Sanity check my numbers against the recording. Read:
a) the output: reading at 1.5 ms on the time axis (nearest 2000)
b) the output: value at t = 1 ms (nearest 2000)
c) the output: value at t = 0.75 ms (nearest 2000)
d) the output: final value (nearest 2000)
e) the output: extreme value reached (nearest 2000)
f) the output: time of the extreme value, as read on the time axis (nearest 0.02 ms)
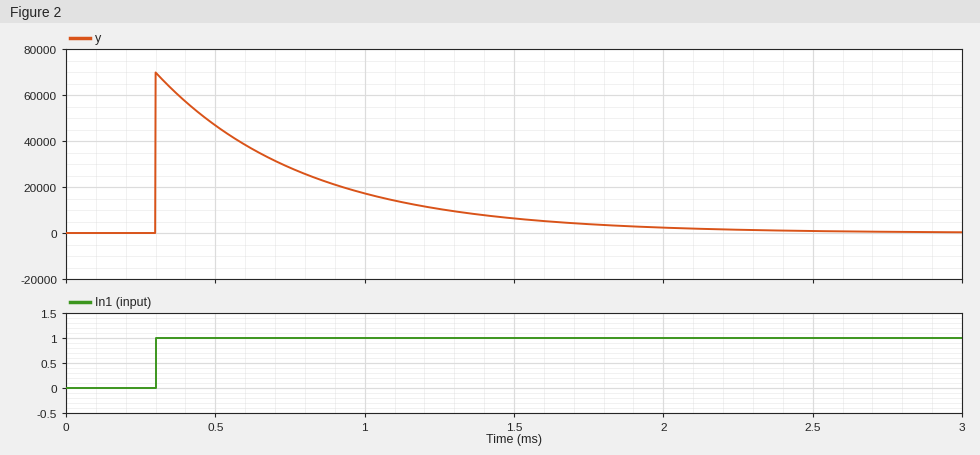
6000
18000
28000
0
70000
0.30 ms
